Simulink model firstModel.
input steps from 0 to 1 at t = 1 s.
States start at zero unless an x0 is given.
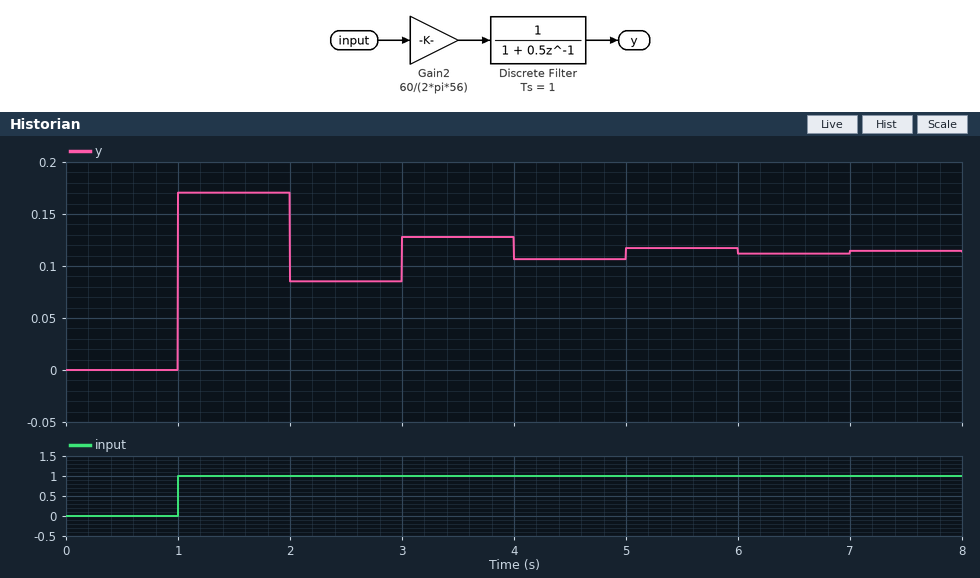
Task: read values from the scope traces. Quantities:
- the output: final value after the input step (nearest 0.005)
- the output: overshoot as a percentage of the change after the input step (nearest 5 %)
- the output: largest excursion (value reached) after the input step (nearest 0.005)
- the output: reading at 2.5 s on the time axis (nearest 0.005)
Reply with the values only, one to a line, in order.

0.115
50 %
0.170
0.085
